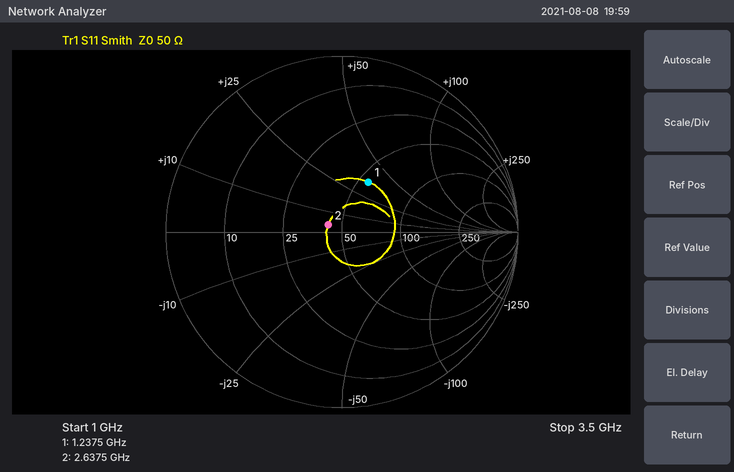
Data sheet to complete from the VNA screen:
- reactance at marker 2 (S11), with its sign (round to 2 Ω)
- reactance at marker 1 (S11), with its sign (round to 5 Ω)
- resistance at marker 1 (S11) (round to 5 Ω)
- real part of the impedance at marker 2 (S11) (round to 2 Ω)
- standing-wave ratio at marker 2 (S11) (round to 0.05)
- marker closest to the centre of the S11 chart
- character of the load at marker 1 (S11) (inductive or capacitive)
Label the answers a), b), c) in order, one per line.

a) +4 Ω
b) +35 Ω
c) 55 Ω
d) 42 Ω
e) 1.20
f) marker 2
g) inductive
